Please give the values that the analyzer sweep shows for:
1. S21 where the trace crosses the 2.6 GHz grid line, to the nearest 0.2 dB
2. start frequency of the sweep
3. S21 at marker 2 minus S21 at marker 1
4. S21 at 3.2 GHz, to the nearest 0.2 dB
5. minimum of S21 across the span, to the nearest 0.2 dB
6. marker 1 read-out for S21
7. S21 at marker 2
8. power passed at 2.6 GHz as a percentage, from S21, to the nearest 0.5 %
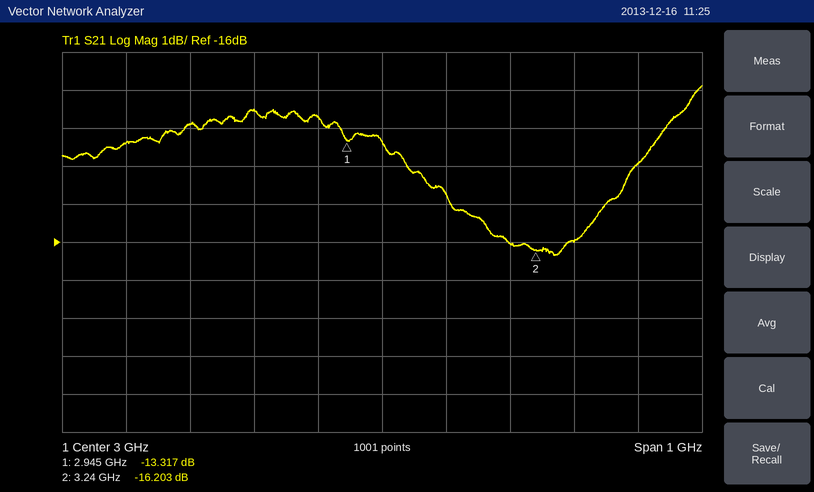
-13.4 dB
2.5 GHz
-2.886 dB
-16.0 dB
-16.4 dB
-13.317 dB
-16.203 dB
4.5 %
